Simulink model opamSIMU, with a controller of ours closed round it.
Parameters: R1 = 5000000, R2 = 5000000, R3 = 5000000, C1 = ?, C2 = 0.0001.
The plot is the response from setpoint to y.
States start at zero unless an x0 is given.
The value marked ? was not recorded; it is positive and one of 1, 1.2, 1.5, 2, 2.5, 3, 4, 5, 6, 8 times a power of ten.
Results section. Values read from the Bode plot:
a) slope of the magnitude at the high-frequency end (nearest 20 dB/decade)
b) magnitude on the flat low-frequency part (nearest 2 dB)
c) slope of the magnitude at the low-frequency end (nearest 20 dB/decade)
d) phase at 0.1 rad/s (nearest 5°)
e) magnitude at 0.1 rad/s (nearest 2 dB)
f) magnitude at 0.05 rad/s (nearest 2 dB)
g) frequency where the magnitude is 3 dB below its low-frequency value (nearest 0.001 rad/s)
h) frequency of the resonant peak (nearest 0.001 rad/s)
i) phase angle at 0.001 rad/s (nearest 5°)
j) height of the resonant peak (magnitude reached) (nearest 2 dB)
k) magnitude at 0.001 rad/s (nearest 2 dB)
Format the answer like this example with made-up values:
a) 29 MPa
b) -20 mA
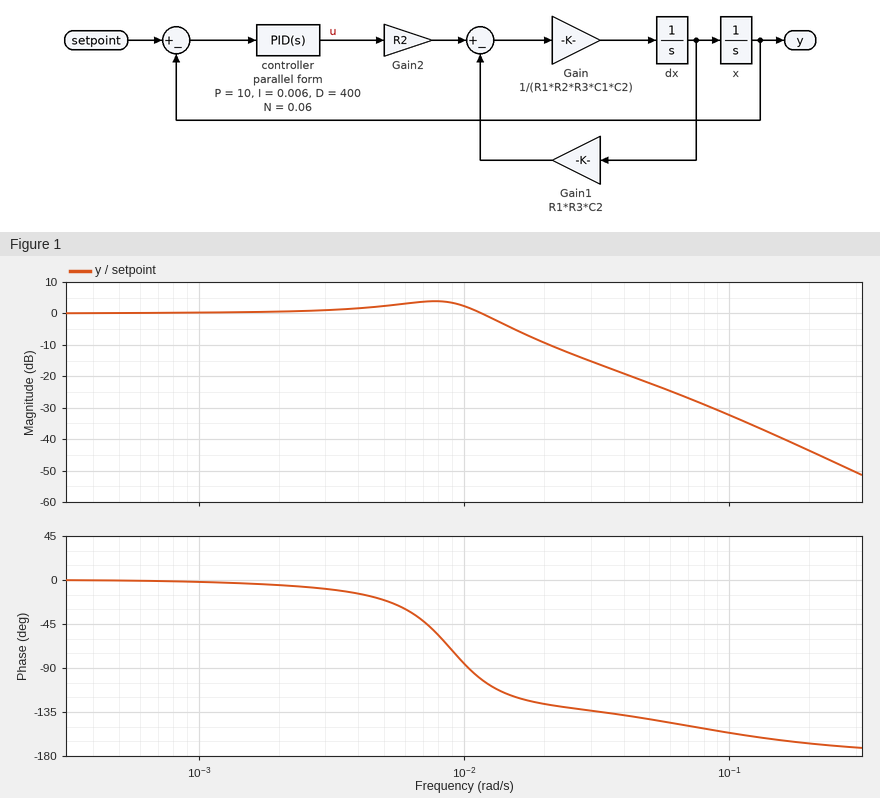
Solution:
a) -40 dB/decade
b) 0 dB
c) 0 dB/decade
d) -155°
e) -32 dB
f) -22 dB
g) 0.014 rad/s
h) 0.008 rad/s
i) 0°
j) 4 dB
k) 0 dB
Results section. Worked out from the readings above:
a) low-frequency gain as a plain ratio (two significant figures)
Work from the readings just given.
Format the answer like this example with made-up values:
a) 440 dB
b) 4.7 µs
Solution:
a) 1.0
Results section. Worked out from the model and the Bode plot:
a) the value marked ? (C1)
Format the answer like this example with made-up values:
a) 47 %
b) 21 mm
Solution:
a) 5e-05
